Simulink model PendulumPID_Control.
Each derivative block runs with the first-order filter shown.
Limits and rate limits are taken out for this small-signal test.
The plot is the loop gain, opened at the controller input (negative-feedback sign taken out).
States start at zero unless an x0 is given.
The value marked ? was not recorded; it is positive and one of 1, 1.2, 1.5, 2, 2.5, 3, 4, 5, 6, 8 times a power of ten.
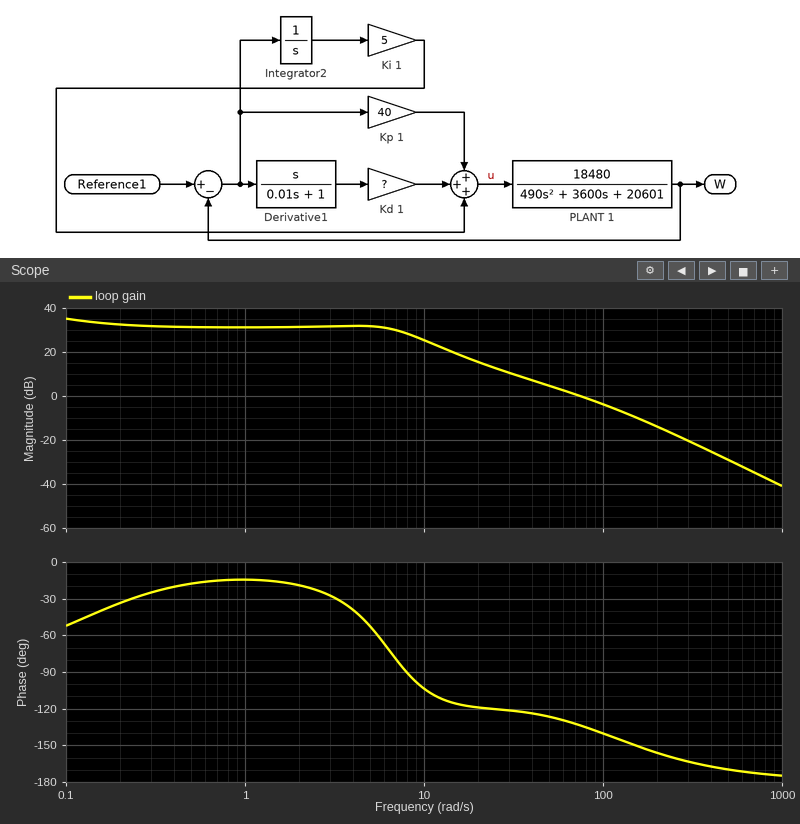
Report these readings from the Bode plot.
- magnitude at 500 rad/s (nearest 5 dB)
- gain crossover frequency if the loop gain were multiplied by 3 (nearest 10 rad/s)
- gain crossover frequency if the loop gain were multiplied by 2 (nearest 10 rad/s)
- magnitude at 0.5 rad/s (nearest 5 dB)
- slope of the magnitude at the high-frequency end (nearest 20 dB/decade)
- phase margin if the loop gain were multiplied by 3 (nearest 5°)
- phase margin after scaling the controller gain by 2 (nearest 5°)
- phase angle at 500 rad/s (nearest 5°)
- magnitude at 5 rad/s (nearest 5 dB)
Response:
-30 dB
150 rad/s
120 rad/s
30 dB
-40 dB/decade
30°
35°
-170°
30 dB
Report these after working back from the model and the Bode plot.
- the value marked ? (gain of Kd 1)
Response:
2
